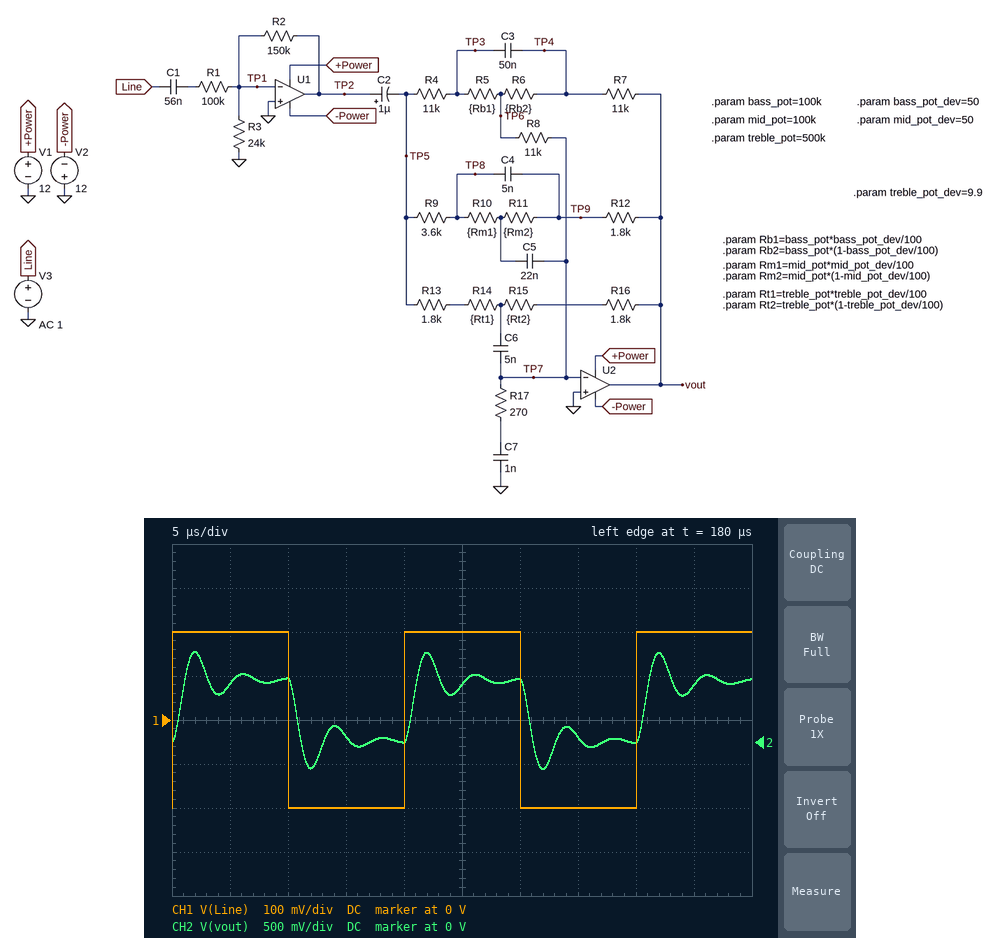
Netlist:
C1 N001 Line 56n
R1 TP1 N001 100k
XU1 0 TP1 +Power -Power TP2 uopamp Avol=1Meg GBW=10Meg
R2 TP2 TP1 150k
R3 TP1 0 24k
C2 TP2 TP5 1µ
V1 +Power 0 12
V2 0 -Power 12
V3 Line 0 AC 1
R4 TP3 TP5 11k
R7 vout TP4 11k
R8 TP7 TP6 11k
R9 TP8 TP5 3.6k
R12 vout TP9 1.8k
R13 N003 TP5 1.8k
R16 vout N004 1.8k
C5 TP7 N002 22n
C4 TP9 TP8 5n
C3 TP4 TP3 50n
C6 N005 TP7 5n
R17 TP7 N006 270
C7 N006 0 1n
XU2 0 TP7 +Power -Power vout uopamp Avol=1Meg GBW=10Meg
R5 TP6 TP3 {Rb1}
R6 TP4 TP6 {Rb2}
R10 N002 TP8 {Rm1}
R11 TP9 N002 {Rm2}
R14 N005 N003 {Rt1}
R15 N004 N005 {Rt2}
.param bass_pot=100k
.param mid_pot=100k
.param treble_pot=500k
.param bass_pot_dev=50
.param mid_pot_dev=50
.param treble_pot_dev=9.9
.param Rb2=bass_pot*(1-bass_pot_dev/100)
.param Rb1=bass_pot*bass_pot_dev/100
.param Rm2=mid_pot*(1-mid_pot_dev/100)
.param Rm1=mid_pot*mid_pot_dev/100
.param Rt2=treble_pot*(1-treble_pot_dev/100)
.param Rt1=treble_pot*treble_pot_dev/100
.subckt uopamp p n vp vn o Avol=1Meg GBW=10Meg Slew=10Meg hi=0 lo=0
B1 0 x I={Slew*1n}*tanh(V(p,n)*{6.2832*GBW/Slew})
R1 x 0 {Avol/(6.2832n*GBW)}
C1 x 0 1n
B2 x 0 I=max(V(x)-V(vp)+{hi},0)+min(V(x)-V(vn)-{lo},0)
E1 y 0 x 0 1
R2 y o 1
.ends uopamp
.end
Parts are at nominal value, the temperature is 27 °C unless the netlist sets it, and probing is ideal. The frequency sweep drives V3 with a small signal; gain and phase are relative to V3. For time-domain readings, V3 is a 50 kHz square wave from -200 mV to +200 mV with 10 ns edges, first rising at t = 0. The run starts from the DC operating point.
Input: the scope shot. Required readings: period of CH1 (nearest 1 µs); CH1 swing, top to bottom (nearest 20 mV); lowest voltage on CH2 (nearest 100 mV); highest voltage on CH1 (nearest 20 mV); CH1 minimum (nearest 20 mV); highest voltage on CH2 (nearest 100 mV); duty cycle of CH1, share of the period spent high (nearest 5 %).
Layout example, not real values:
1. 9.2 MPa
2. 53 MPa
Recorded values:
1. 20 µs
2. 400 mV
3. -300 mV
4. 200 mV
5. -200 mV
6. 1.0 V
7. 50 %
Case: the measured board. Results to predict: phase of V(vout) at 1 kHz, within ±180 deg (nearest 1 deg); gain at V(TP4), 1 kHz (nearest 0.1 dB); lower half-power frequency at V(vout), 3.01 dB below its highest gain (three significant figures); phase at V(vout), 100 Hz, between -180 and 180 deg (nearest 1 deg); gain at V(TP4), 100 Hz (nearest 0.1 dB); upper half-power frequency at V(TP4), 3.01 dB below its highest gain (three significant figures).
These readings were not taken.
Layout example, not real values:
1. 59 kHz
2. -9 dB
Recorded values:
1. 7 deg
2. -9.2 dB
3. 166 kHz
4. 27 deg
5. 0.1 dB
6. 358 kHz
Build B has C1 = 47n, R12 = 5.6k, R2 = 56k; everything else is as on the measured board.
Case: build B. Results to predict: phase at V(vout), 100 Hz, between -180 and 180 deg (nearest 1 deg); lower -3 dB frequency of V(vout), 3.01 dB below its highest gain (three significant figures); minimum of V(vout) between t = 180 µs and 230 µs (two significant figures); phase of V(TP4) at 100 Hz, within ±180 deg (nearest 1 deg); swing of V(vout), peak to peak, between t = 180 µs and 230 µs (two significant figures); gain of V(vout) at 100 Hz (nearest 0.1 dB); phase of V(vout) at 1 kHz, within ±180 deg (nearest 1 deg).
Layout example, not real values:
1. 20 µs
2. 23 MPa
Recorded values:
1. 31 deg
2. 153 kHz
3. -300 mV
4. 4 deg
5. 870 mV
6. -5.3 dB
7. 14 deg
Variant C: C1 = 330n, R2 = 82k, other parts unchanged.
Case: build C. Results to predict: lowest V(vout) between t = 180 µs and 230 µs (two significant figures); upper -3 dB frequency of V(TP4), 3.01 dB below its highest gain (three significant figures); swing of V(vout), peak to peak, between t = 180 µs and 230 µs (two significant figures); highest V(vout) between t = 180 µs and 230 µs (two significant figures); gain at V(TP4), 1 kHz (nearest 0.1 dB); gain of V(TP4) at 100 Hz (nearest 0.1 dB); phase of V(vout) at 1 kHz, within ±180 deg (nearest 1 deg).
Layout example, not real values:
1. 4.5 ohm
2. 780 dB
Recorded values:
1. -160 mV
2. 362 kHz
3. 730 mV
4. 570 mV
5. -14.4 dB
6. -4.8 dB
7. 6 deg
